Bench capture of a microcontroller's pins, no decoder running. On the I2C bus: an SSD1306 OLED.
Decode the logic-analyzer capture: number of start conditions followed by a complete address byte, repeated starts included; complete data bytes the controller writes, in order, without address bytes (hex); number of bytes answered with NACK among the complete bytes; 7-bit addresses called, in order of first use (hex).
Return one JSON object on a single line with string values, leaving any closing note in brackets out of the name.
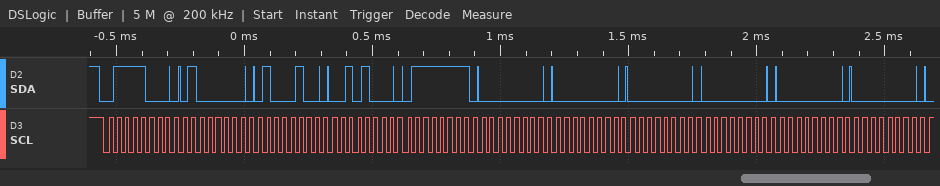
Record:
{"number of start conditions followed by a complete address byte, repeated starts included": "1", "complete data bytes the controller writes, in order, without address bytes": "40 44 28 7F 00 00 00 00 00 00", "number of bytes answered with NACK among the complete bytes": "0", "7-bit addresses called, in order of first use": "0x3C"}
